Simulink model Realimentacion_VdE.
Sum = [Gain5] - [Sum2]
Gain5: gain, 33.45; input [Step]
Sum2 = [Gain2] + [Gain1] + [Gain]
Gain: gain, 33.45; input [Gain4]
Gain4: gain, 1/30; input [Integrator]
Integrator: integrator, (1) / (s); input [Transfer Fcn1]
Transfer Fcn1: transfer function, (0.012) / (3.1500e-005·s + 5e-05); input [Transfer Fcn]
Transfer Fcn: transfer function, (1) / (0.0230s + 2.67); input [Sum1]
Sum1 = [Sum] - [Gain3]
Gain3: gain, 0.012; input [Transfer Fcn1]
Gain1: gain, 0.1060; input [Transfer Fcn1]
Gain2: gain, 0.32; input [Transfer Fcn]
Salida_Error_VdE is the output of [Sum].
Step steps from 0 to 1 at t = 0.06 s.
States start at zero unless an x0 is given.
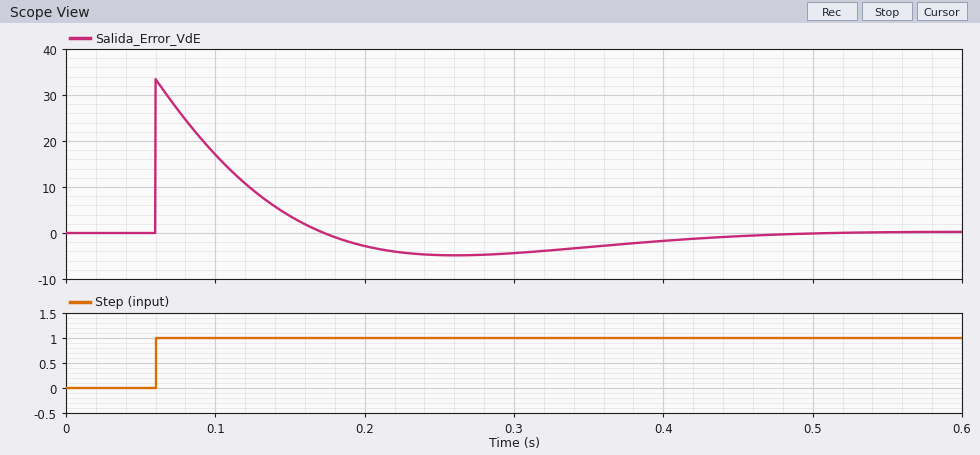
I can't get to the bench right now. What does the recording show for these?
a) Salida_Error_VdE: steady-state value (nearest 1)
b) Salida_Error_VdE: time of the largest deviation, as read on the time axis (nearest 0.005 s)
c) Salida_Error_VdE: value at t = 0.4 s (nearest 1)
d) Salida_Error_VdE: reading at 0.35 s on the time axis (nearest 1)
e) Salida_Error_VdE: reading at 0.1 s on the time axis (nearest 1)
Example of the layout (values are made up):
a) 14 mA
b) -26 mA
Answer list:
a) 0
b) 0.060 s
c) -2
d) -3
e) 17
